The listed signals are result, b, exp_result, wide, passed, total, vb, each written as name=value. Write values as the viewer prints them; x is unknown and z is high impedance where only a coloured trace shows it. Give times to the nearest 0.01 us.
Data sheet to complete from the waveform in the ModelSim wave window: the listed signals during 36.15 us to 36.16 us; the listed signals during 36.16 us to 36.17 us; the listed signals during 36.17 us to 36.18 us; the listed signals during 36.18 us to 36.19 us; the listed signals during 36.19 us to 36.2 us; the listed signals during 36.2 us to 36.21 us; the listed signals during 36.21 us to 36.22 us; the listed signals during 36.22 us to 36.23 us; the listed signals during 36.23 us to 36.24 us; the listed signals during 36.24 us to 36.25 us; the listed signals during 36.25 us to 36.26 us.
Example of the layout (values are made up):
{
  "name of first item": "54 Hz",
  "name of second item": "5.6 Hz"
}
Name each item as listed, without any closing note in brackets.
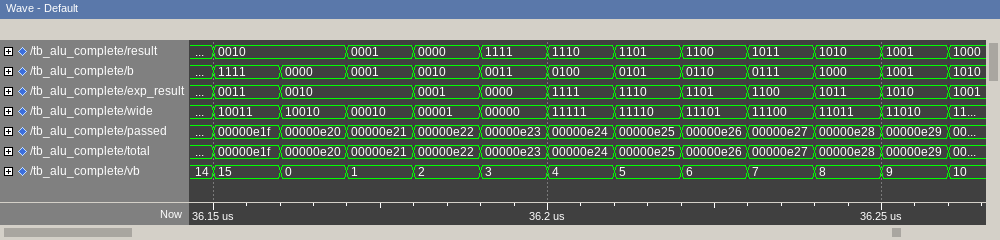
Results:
{
  "the listed signals during 36.15 us to 36.16 us": "result=0010, b=1111, exp_result=0011, wide=10011, passed=00000e1f, total=00000e1f, vb=15",
  "the listed signals during 36.16 us to 36.17 us": "result=0010, b=0000, exp_result=0010, wide=10010, passed=00000e20, total=00000e20, vb=0",
  "the listed signals during 36.17 us to 36.18 us": "result=0001, b=0001, exp_result=0010, wide=00010, passed=00000e21, total=00000e21, vb=1",
  "the listed signals during 36.18 us to 36.19 us": "result=0000, b=0010, exp_result=0001, wide=00001, passed=00000e22, total=00000e22, vb=2",
  "the listed signals during 36.19 us to 36.2 us": "result=1111, b=0011, exp_result=0000, wide=00000, passed=00000e23, total=00000e23, vb=3",
  "the listed signals during 36.2 us to 36.21 us": "result=1110, b=0100, exp_result=1111, wide=11111, passed=00000e24, total=00000e24, vb=4",
  "the listed signals during 36.21 us to 36.22 us": "result=1101, b=0101, exp_result=1110, wide=11110, passed=00000e25, total=00000e25, vb=5",
  "the listed signals during 36.22 us to 36.23 us": "result=1100, b=0110, exp_result=1101, wide=11101, passed=00000e26, total=00000e26, vb=6",
  "the listed signals during 36.23 us to 36.24 us": "result=1011, b=0111, exp_result=1100, wide=11100, passed=00000e27, total=00000e27, vb=7",
  "the listed signals during 36.24 us to 36.25 us": "result=1010, b=1000, exp_result=1011, wide=11011, passed=00000e28, total=00000e28, vb=8",
  "the listed signals during 36.25 us to 36.26 us": "result=1001, b=1001, exp_result=1010, wide=11010, passed=00000e29, total=00000e29, vb=9"
}
